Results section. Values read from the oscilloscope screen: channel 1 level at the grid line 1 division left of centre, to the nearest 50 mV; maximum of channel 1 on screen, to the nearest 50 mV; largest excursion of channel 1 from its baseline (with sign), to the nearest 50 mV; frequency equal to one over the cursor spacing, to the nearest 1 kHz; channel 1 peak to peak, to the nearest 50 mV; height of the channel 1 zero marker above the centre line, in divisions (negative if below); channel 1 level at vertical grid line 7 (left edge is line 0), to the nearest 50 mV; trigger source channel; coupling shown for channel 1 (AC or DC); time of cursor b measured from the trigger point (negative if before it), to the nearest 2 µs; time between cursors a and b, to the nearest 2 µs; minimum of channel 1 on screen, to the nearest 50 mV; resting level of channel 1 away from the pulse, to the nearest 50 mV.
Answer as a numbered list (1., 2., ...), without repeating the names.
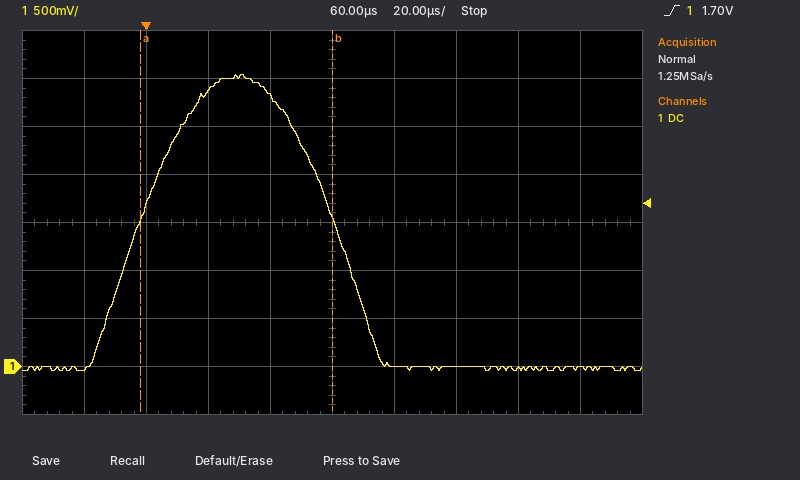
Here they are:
1. 2.80 V
2. 3.05 V
3. +3.05 V
4. 16 kHz
5. 3.10 V
6. -3.0 div
7. 0 mV
8. channel 1
9. DC
10. +60 µs
11. 62 µs
12. -50 mV
13. 0 mV
